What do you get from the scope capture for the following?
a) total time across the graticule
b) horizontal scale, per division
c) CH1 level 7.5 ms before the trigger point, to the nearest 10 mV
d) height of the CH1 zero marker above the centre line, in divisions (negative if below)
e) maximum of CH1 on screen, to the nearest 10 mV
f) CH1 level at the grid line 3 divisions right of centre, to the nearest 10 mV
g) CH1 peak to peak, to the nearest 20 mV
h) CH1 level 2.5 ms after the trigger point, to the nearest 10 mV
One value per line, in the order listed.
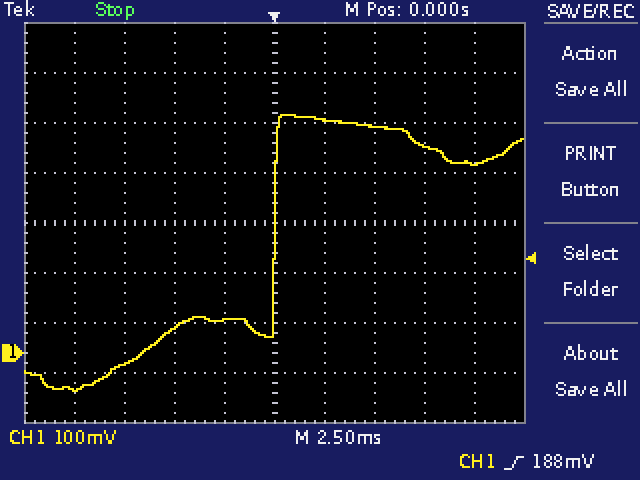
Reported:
25 ms
2.5 ms
-20 mV
-2.6 div
480 mV
410 mV
560 mV
470 mV
